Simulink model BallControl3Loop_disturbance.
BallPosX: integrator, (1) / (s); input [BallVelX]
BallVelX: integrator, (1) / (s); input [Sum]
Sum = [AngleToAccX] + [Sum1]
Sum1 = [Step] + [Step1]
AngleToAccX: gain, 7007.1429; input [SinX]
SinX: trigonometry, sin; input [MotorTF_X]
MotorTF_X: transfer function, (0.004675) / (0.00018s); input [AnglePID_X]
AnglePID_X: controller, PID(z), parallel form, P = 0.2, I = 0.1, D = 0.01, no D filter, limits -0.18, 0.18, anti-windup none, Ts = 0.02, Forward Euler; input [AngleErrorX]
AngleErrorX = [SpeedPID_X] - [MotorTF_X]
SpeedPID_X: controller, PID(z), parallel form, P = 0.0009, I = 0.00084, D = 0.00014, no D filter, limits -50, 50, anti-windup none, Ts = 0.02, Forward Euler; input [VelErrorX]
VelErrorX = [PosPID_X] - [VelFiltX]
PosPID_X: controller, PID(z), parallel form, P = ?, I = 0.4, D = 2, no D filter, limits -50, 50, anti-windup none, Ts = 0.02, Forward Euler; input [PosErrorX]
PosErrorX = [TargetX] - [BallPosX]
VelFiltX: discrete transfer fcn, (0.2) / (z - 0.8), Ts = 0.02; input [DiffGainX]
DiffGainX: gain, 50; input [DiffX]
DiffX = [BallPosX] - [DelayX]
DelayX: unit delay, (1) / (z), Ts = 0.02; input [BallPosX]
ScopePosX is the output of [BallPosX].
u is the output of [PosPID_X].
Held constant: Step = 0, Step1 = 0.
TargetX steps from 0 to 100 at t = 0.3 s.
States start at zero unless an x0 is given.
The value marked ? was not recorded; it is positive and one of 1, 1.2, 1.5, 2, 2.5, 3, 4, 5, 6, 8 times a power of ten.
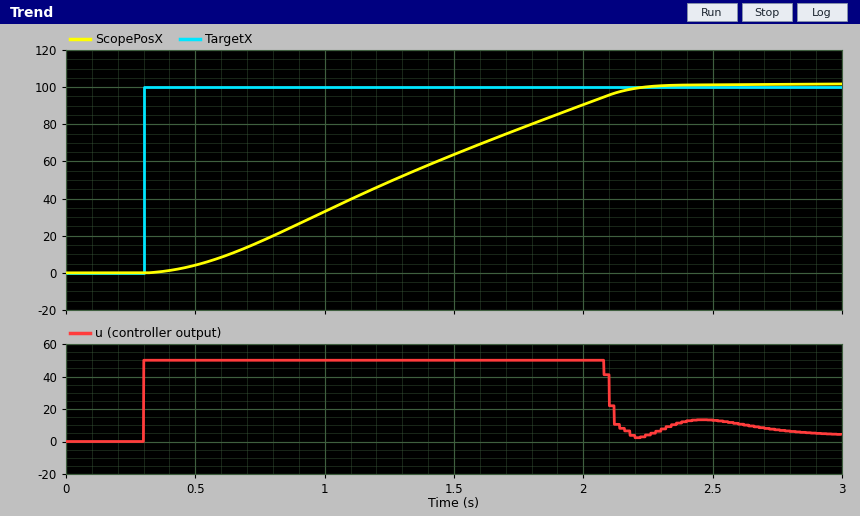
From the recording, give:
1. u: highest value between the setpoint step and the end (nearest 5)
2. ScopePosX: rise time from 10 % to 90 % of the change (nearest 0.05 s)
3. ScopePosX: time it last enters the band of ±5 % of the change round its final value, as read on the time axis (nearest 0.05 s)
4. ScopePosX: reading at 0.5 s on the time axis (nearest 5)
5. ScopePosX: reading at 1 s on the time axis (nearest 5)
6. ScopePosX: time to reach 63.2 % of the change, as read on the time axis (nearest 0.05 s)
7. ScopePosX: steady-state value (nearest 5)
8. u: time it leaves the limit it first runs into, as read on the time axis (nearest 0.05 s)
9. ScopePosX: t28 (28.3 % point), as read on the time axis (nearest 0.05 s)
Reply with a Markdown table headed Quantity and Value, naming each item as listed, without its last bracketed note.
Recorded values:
| Quantity | Value |
|---|---|
| u: highest value between the setpoint step and the end | 50 |
| ScopePosX: rise time from 10 % to 90 % of the change | 1.40 s |
| ScopePosX: time it last enters the band of ±5 % of the change round its final value, as read on the time axis | 2.10 s |
| ScopePosX: reading at 0.5 s on the time axis | 5 |
| ScopePosX: reading at 1 s on the time axis | 35 |
| ScopePosX: time to reach 63.2 % of the change, as read on the time axis | 1.50 s |
| ScopePosX: steady-state value | 100 |
| u: time it leaves the limit it first runs into, as read on the time axis | 2.10 s |
| ScopePosX: t28 (28.3 % point), as read on the time axis | 0.95 s |
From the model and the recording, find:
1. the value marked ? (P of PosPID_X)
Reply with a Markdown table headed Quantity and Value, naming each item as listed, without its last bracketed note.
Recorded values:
| Quantity | Value |
|---|---|
| the value marked ? | 20 |
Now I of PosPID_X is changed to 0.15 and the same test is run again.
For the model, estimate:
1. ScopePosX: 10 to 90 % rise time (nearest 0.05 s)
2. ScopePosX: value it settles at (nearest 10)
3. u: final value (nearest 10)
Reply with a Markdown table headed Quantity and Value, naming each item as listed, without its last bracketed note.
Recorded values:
| Quantity | Value |
|---|---|
| ScopePosX: 10 to 90 % rise time | 1.35 s |
| ScopePosX: value it settles at | 100 |
| u: final value | 0 |
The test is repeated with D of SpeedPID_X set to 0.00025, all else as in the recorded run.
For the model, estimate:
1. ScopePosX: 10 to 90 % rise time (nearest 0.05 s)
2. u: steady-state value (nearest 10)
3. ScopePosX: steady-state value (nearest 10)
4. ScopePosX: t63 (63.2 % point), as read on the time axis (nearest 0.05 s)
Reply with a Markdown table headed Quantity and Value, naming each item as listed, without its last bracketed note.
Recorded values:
| Quantity | Value |
|---|---|
| ScopePosX: 10 to 90 % rise time | 1.35 s |
| u: steady-state value | 0 |
| ScopePosX: steady-state value | 100 |
| ScopePosX: t63 (63.2 % point), as read on the time axis | 1.55 s |
